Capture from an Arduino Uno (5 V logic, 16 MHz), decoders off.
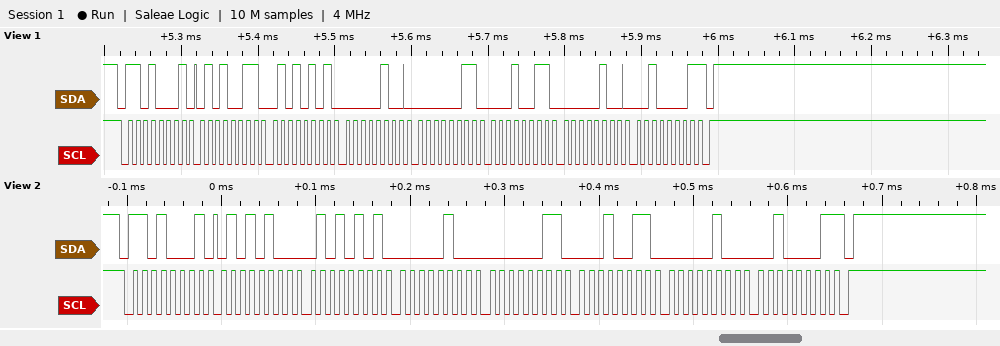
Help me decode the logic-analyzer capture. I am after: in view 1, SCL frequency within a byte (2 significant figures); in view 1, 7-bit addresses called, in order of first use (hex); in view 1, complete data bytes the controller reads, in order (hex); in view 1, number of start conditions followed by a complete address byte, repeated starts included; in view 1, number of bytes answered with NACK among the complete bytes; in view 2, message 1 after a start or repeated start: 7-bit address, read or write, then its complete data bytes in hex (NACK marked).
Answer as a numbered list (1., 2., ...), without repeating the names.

1. 100 kHz
2. 0x68
3. 53 55 04 03 13 04 21
4. 1
5. 1
6. 0x68 read: 54 55 04 03 13 04 21 NACK
